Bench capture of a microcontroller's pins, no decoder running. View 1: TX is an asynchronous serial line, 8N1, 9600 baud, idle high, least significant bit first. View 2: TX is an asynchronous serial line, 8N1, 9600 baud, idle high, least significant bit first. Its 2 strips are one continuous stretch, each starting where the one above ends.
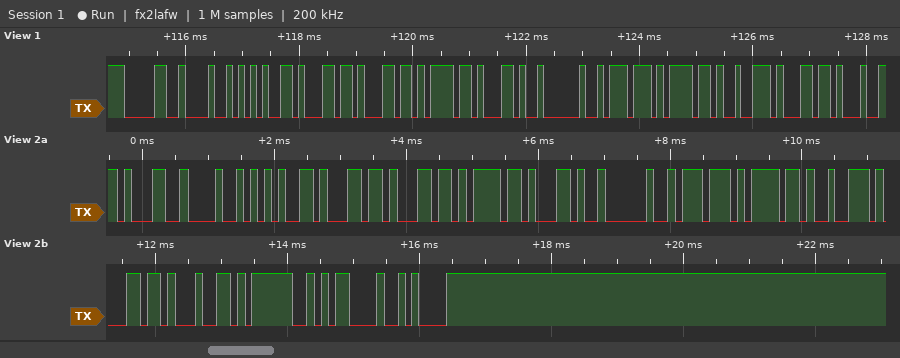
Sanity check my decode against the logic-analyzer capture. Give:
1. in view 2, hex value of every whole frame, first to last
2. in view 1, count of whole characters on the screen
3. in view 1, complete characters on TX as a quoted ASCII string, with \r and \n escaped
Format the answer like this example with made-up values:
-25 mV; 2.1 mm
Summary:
31 48 65 6C 6C 6F 2C 20 77 6F 72 6C 64 3F 0D 0A; 12; "0Hello, worl"
